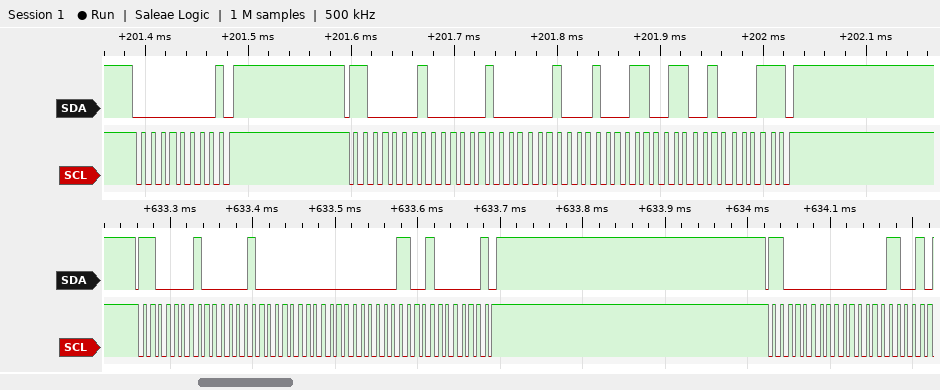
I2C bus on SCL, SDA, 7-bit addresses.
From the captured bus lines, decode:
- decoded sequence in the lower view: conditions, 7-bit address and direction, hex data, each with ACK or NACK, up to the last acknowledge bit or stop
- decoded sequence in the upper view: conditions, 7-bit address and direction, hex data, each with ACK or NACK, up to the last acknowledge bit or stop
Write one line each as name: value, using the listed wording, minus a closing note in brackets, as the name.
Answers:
decoded sequence in the lower view: conditions, 7-bit address and direction, hex data, each with ACK or NACK, up to the last acknowledge bit or stop: start, address 60 read ACK, 04 ACK, 00 ACK, 03 ACK, 40 NACK, stop, start, address 60 write ACK, 03 ACK
decoded sequence in the upper view: conditions, 7-bit address and direction, hex data, each with ACK or NACK, up to the last acknowledge bit or stop: start, address 00 write NACK, stop, start, address 60 read ACK, 04 ACK, 11 ACK, 33 ACK, 43 NACK, stop
